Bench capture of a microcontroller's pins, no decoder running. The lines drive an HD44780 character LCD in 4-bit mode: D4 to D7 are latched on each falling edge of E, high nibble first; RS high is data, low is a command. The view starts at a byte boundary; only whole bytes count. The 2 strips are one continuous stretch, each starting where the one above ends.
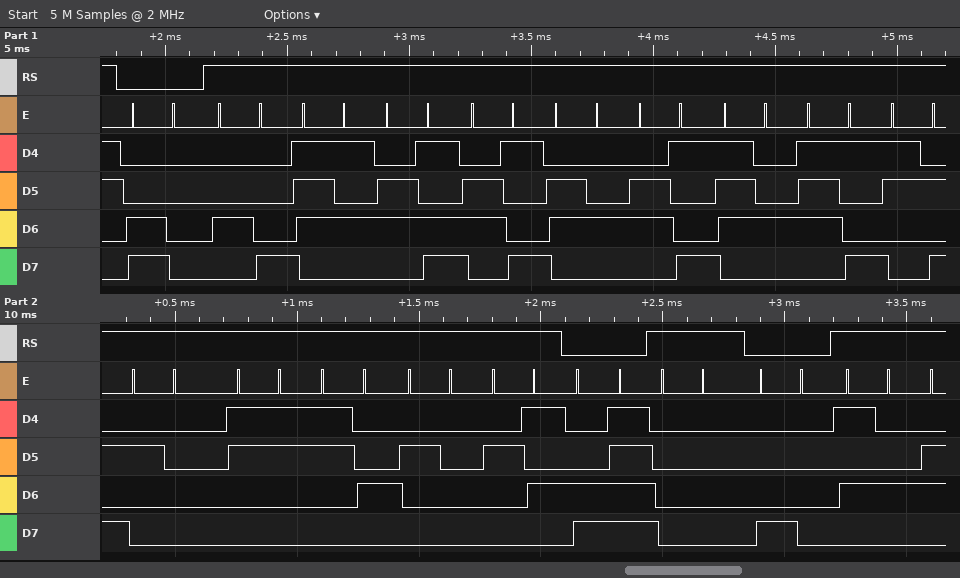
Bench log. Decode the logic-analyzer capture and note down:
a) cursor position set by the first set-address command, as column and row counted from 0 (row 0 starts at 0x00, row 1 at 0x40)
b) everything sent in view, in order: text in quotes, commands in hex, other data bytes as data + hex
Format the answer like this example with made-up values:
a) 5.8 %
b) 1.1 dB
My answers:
a) column 0, row 1
b) 0xC0 "Humidity: 34 %" 0xCF data 00 0x80 "T"
